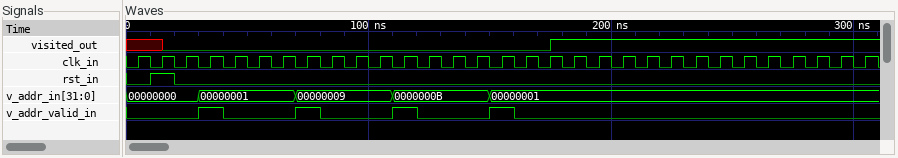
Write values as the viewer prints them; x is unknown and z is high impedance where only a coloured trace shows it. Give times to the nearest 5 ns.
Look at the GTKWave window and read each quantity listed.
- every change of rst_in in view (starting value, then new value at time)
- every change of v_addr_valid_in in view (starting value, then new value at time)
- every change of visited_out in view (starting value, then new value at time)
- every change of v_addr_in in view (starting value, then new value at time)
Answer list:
0, 1 at 10 ns, 0 at 20 ns
0, 1 at 30 ns, 0 at 40 ns, 1 at 70 ns, 0 at 80 ns, 1 at 110 ns, 0 at 120 ns, 1 at 150 ns, 0 at 160 ns
x, 0 at 15 ns, 1 at 175 ns
00000000, 00000001 at 30 ns, 00000009 at 70 ns, 0000000B at 110 ns, 00000001 at 150 ns
